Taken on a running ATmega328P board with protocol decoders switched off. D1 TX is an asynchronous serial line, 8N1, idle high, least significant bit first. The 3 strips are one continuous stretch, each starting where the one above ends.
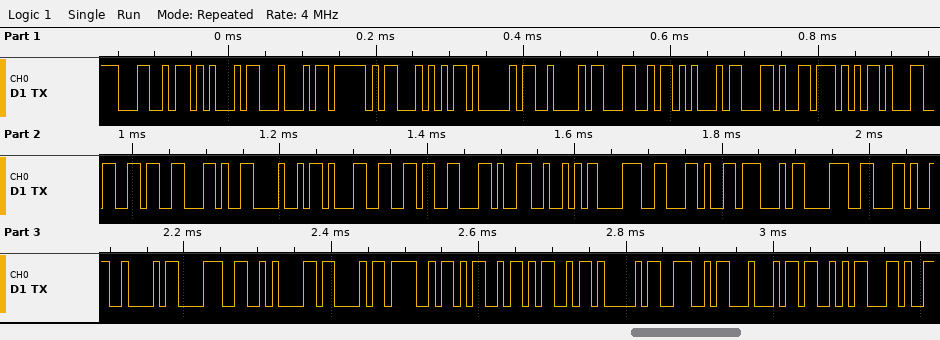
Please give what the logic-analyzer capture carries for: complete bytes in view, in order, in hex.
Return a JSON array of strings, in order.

["4C 45 44 5F 54 41 42 4C 45 2C 57 31 36 2C 48 31 36 2C 52 38 2C 47 38 2C 42 38 0A 43 4F 4D 4D 41 4E 44 53 2C"]
